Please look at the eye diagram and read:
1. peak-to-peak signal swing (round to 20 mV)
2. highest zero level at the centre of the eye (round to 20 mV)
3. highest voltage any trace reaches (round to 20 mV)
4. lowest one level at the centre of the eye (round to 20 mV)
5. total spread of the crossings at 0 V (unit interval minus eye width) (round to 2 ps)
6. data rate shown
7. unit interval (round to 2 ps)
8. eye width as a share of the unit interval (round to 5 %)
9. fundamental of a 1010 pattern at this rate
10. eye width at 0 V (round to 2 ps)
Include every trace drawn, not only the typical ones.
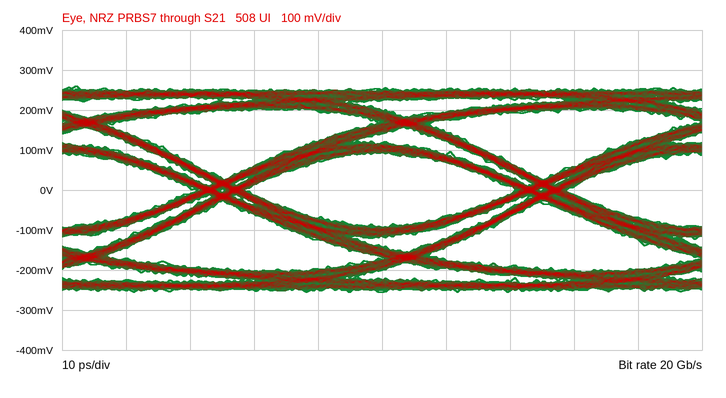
520 mV
-100 mV
260 mV
100 mV
8 ps
20 Gb/s
50 ps
85 %
10 GHz
42 ps
